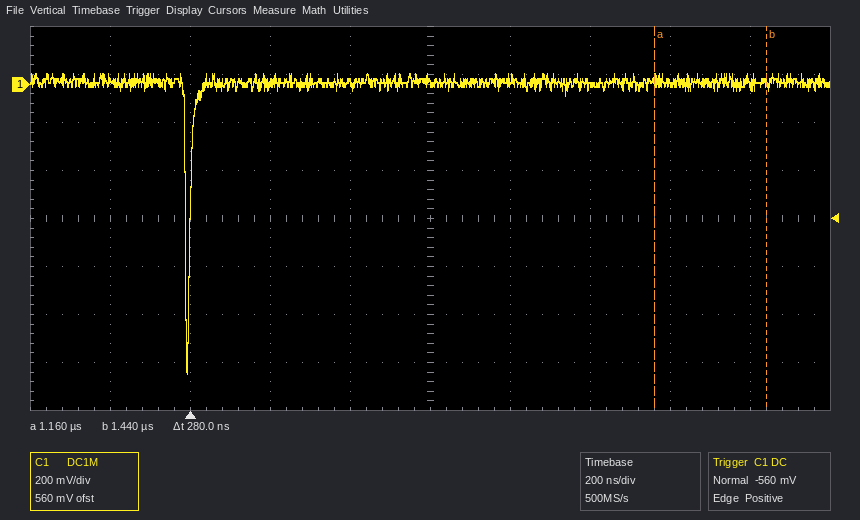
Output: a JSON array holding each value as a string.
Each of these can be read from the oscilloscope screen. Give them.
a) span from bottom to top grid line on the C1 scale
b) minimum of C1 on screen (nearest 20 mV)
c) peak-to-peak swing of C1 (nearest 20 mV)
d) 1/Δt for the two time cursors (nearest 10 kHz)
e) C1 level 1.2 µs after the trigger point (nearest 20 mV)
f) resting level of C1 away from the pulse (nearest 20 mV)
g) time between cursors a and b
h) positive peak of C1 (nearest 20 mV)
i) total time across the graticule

["1.6 V", "-1.20 V", "1.24 V", "3.57 MHz", "0 mV", "0 mV", "280 ns", "40 mV", "2 µs"]
